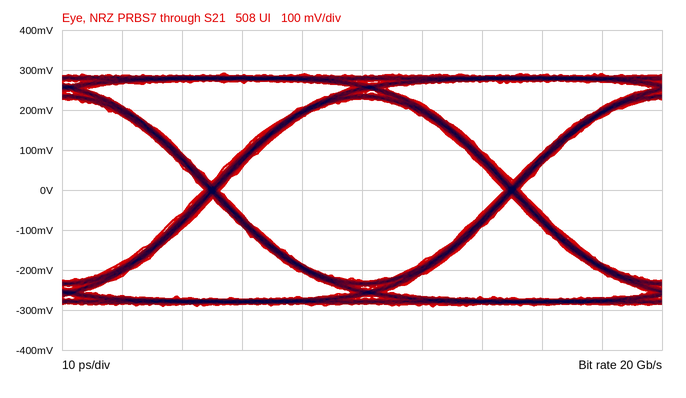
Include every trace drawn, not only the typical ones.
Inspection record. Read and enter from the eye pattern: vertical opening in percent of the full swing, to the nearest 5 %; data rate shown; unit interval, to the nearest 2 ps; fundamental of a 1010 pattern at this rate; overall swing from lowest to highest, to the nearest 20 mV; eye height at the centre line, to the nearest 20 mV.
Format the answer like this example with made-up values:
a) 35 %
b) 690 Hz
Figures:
a) 80 %
b) 20 Gb/s
c) 50 ps
d) 10 GHz
e) 580 mV
f) 460 mV
